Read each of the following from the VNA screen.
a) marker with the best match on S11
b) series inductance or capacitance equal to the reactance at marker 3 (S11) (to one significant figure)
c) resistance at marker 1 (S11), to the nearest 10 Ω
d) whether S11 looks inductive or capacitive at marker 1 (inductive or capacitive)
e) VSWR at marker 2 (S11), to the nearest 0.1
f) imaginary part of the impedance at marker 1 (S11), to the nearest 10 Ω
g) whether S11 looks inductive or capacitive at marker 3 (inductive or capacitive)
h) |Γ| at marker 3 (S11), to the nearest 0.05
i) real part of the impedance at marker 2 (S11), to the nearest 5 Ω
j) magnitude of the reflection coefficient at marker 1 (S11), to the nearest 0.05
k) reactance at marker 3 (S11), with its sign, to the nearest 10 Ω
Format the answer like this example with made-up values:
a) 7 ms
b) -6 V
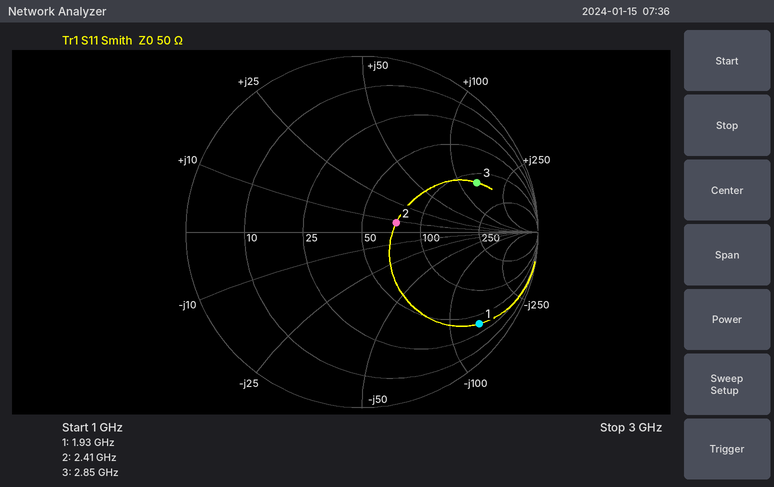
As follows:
a) marker 2
b) 8 nH
c) 40 Ω
d) capacitive
e) 1.5
f) -140 Ω
g) inductive
h) 0.70
i) 75 Ω
j) 0.85
k) +140 Ω
